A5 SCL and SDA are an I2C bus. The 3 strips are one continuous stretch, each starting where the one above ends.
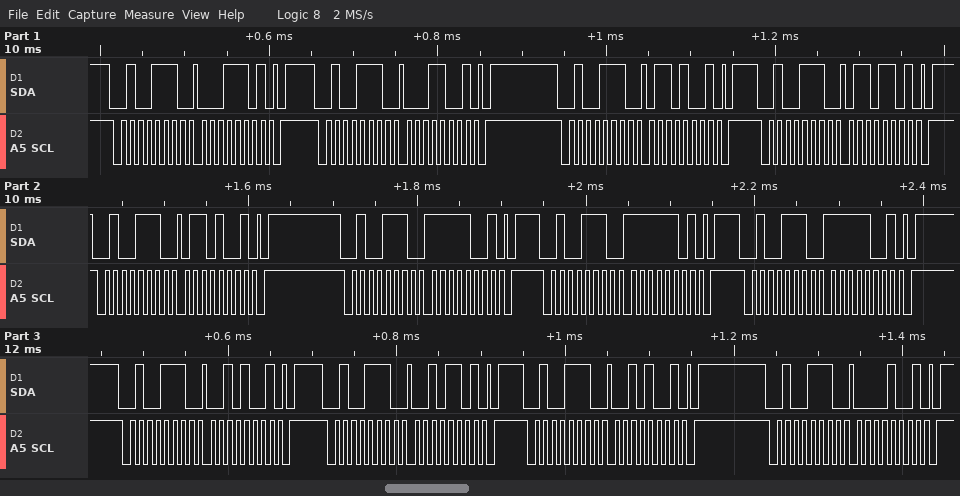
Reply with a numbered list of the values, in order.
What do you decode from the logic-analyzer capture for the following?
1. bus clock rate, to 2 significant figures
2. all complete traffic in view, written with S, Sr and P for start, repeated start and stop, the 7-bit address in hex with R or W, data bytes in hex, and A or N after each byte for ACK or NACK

1. 100 kHz
2. S 27W A 1D A P S 27W A 19 A P S 27W A 69 A P S 27W A 6D A P S 27W A 69 A P S 27W A F9 A P S 27W A FD A P S 27W A F9 A P S 27W A 29 A P S 27W A 2D A P S 27W A 29 A P S 27W A 09 A P
